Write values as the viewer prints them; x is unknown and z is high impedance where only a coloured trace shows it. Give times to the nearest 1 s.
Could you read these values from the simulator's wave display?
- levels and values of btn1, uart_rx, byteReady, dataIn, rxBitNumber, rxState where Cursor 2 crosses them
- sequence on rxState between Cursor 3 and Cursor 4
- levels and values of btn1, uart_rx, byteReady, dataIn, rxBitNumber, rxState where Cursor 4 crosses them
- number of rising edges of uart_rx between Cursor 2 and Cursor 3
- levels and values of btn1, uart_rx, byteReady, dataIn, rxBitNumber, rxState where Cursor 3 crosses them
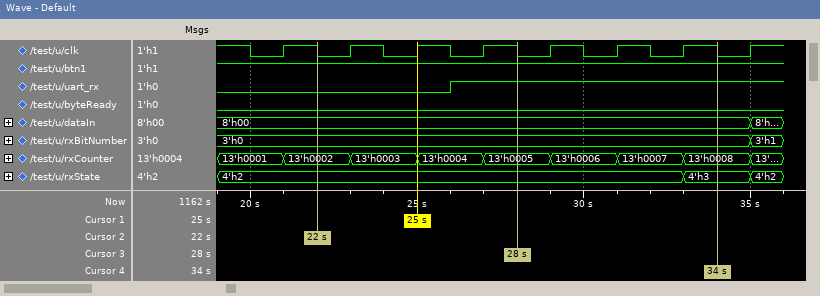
btn1=1, uart_rx=0, byteReady=0, dataIn=8'h00, rxBitNumber=3'h0, rxState=4'h2
4'h2, 4'h3
btn1=1, uart_rx=1, byteReady=0, dataIn=8'h00, rxBitNumber=3'h0, rxState=4'h3
1
btn1=1, uart_rx=1, byteReady=0, dataIn=8'h00, rxBitNumber=3'h0, rxState=4'h2
